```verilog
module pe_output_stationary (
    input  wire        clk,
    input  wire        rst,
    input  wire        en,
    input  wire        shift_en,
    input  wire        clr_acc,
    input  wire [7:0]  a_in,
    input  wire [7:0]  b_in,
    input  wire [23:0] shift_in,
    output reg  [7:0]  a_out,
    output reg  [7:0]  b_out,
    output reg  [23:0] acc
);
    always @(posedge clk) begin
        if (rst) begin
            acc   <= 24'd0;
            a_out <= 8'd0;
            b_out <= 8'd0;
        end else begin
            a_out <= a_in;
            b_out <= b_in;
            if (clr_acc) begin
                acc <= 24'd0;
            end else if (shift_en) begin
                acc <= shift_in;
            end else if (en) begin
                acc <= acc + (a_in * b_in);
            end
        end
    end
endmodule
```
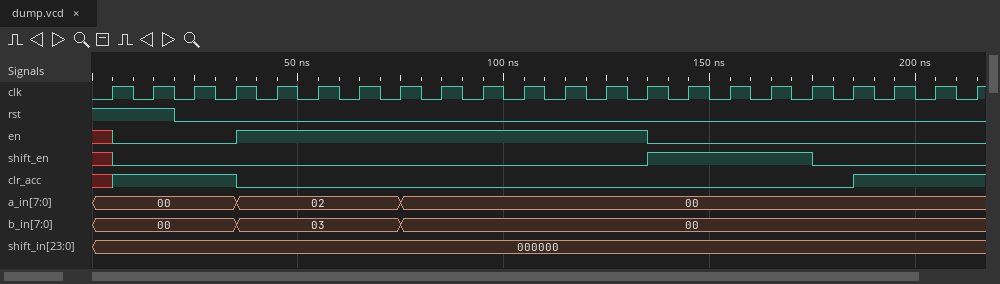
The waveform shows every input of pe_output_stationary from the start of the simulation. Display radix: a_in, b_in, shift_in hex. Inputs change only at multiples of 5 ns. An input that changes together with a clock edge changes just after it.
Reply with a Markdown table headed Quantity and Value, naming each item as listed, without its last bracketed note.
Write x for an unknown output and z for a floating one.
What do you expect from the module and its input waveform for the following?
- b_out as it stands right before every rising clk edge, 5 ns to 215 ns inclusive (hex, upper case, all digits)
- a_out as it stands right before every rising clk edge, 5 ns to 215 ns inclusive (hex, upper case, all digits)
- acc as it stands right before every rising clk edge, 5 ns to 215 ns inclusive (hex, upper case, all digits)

| Quantity | Value |
|---|---|
| b_out as it stands right before every rising clk edge, 5 ns to 215 ns inclusive | x, 00, 00, 00, 00, 03, 03, 03, 03, 00, 00, 00, 00, 00, 00, 00, 00, 00, 00, 00, 00, 00 |
| a_out as it stands right before every rising clk edge, 5 ns to 215 ns inclusive | x, 00, 00, 00, 00, 02, 02, 02, 02, 00, 00, 00, 00, 00, 00, 00, 00, 00, 00, 00, 00, 00 |
| acc as it stands right before every rising clk edge, 5 ns to 215 ns inclusive | x, 000000, 000000, 000000, 000000, 000006, 00000C, 000012, 000018, 000018, 000018, 000018, 000018, 000018, 000018, 000000, 000000, 000000, 000000, 000000, 000000, 000000 |
